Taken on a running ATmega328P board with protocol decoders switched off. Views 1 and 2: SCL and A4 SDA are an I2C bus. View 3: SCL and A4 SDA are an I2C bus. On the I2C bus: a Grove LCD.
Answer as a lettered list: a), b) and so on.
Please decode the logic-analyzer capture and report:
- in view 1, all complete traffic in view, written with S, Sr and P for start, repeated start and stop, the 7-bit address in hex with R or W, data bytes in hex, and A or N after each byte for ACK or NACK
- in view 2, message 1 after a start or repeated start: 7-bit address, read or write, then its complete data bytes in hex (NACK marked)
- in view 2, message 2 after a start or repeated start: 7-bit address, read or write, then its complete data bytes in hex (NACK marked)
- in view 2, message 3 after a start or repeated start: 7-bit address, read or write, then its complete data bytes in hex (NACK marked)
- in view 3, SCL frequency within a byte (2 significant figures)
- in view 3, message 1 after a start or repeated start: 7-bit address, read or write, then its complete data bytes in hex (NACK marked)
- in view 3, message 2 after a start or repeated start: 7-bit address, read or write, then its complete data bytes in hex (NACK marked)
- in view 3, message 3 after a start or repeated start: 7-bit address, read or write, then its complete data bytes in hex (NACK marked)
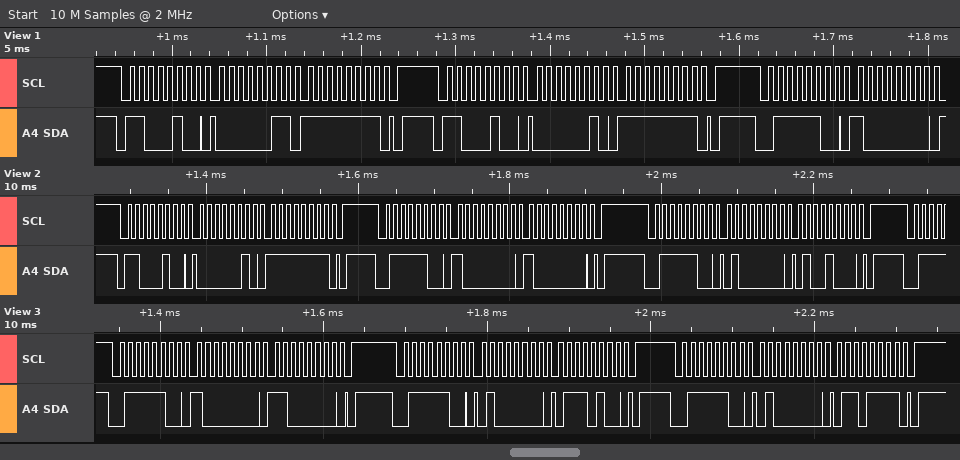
a) S 62W A 03 A FF A P S 62W A 02 A FF A P S 3EW A 80 A
b) 0x62 write: 02 FF
c) 0x3E write: 80 80
d) 0x3E write: 40 48
e) 100 kHz
f) 0x3E write: 80 C0
g) 0x3E write: 40 74
h) 0x3E write: 40 6F
